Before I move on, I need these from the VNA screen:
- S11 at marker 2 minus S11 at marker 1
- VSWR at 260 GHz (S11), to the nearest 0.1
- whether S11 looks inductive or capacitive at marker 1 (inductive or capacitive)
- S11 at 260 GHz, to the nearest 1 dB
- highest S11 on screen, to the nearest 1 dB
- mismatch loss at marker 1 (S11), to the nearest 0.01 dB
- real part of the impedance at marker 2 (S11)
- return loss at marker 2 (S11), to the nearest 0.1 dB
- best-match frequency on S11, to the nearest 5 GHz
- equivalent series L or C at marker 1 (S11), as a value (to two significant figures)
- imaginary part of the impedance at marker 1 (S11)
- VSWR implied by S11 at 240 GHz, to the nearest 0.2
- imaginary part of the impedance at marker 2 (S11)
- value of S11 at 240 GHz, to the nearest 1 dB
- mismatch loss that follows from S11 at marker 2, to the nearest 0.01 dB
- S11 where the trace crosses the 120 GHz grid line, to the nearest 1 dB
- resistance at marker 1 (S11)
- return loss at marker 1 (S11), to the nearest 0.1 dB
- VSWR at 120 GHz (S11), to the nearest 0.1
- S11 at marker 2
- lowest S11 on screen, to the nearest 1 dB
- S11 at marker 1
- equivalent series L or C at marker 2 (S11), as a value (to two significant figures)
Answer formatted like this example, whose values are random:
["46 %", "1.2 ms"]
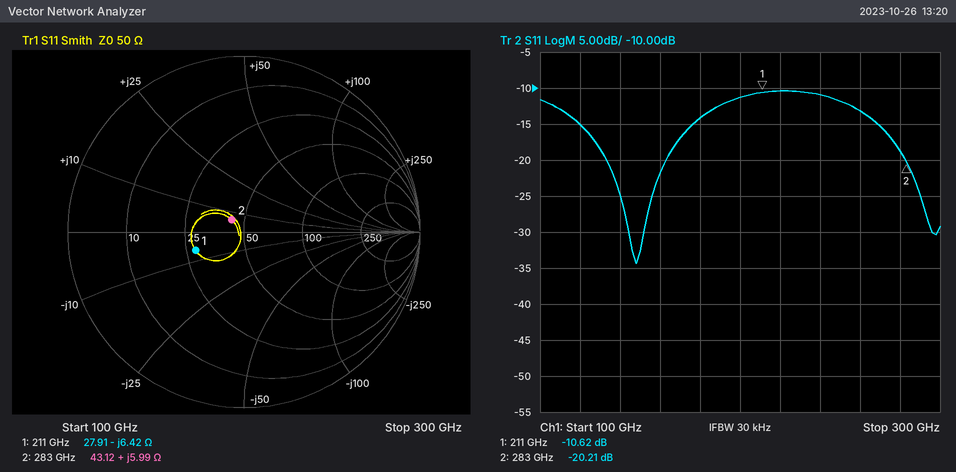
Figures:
["-9.59 dB", "1.6", "capacitive", "-13 dB", "-10 dB", "0.39 dB", "43.12 Ω", "20.2 dB", "150 GHz", "120 fF", "-6.42 Ω", "1.8", "+5.99 Ω", "-11 dB", "0.04 dB", "-15 dB", "27.91 Ω", "10.6 dB", "1.4", "-20.21 dB", "-34 dB", "-10.62 dB", "3.4 pH"]
